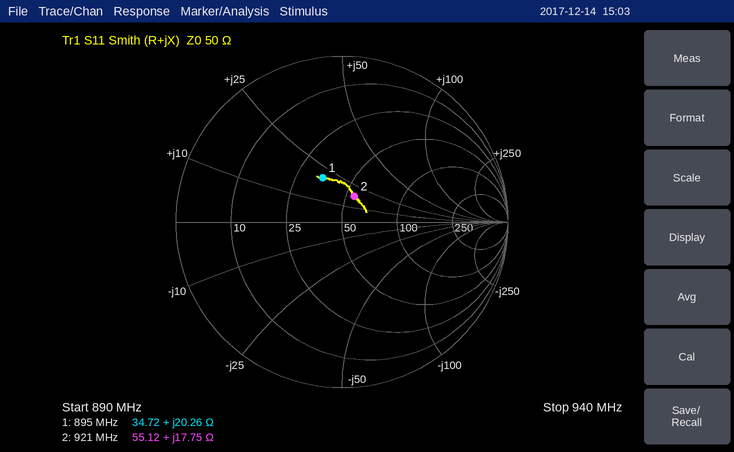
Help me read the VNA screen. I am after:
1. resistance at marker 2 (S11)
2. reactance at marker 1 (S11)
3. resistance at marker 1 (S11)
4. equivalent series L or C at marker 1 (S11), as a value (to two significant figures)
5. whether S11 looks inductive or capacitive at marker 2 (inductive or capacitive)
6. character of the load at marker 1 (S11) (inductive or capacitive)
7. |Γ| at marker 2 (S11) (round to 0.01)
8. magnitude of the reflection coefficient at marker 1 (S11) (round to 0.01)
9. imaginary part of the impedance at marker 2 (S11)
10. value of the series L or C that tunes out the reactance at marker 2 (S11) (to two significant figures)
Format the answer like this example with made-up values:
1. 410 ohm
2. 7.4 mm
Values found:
1. 55.12 Ω
2. +20.26 Ω
3. 34.72 Ω
4. 3.6 nH
5. inductive
6. inductive
7. 0.17
8. 0.29
9. +17.75 Ω
10. 9.7 pF
